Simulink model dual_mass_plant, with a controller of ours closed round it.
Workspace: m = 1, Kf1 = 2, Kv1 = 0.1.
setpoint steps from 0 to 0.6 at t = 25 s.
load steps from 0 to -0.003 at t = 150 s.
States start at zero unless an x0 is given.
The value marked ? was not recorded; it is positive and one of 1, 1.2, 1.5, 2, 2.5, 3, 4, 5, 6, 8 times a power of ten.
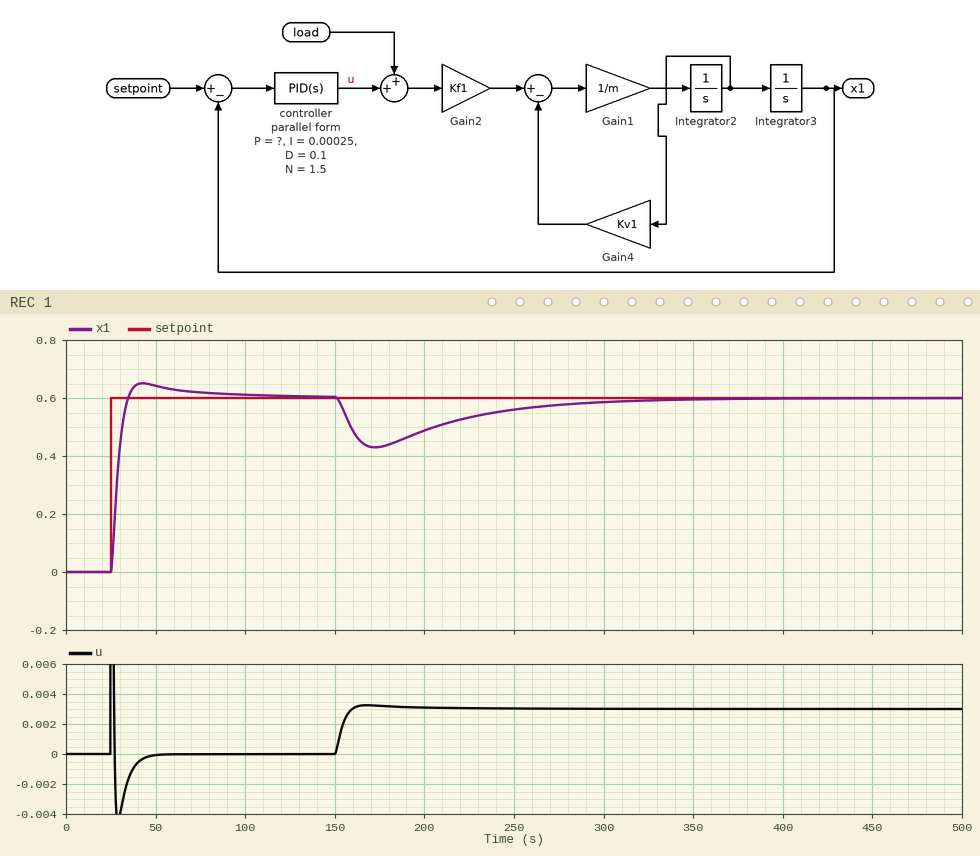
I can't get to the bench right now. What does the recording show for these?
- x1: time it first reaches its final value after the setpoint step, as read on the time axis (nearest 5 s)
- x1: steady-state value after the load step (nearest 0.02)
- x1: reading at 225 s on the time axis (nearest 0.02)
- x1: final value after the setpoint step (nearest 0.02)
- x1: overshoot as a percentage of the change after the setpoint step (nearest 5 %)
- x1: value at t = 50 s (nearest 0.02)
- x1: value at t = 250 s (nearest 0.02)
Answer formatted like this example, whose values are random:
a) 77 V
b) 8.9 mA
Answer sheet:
a) 35 s
b) 0.60
c) 0.54
d) 0.60
e) 10 %
f) 0.64
g) 0.56
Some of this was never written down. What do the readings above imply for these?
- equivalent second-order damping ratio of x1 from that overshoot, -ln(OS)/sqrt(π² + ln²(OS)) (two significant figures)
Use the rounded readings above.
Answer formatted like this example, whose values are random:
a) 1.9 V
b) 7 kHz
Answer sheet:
a) 0.59
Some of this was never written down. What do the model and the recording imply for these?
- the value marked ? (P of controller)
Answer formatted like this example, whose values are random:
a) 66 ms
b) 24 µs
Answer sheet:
a) 0.015
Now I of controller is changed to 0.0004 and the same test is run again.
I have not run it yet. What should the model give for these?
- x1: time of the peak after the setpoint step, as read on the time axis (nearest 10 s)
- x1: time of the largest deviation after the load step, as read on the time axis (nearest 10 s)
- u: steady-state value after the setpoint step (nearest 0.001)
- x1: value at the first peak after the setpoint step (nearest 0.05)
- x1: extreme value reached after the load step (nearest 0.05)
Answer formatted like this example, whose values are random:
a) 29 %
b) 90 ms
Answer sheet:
a) 40 s
b) 170 s
c) 0.000
d) 0.65
e) 0.45
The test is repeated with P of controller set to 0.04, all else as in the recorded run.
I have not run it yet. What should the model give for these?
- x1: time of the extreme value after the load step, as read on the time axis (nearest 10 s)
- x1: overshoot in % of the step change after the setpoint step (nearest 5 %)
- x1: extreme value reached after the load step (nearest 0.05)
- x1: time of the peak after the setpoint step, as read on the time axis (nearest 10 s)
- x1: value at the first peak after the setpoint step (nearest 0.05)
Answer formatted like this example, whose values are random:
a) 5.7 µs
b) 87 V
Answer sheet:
a) 160 s
b) 25 %
c) 0.50
d) 30 s
e) 0.75
